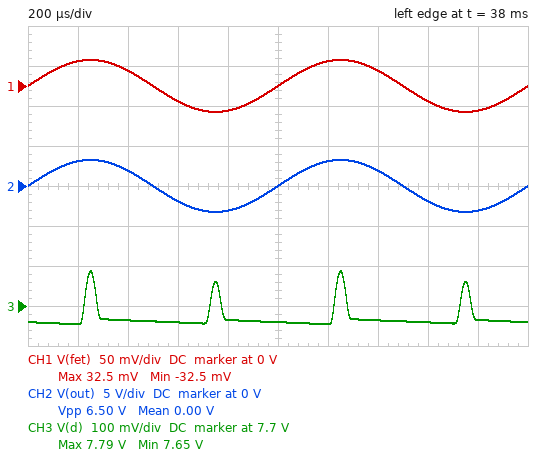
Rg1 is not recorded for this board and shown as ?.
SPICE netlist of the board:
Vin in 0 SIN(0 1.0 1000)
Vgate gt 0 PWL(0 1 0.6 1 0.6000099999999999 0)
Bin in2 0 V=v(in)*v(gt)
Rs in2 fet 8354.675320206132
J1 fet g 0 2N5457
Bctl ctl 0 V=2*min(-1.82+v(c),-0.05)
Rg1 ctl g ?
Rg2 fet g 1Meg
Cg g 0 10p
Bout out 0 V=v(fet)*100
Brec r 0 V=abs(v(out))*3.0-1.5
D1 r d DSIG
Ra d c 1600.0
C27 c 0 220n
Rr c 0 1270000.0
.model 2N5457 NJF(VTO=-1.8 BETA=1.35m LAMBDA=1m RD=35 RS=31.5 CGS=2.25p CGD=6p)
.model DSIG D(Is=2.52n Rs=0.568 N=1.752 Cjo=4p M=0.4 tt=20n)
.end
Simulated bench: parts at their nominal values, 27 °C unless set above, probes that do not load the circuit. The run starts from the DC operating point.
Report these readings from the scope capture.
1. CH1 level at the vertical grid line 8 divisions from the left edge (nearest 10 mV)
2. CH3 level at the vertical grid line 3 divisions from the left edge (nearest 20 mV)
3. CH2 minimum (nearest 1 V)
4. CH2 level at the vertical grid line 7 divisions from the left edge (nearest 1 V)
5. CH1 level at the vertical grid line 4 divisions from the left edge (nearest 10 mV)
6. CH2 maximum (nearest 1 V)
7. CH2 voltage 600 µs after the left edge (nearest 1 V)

-20 mV
7.66 V
-3 V
2 V
-30 mV
3 V
-2 V
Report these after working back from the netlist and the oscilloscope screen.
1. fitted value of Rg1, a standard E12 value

470 kΩ
